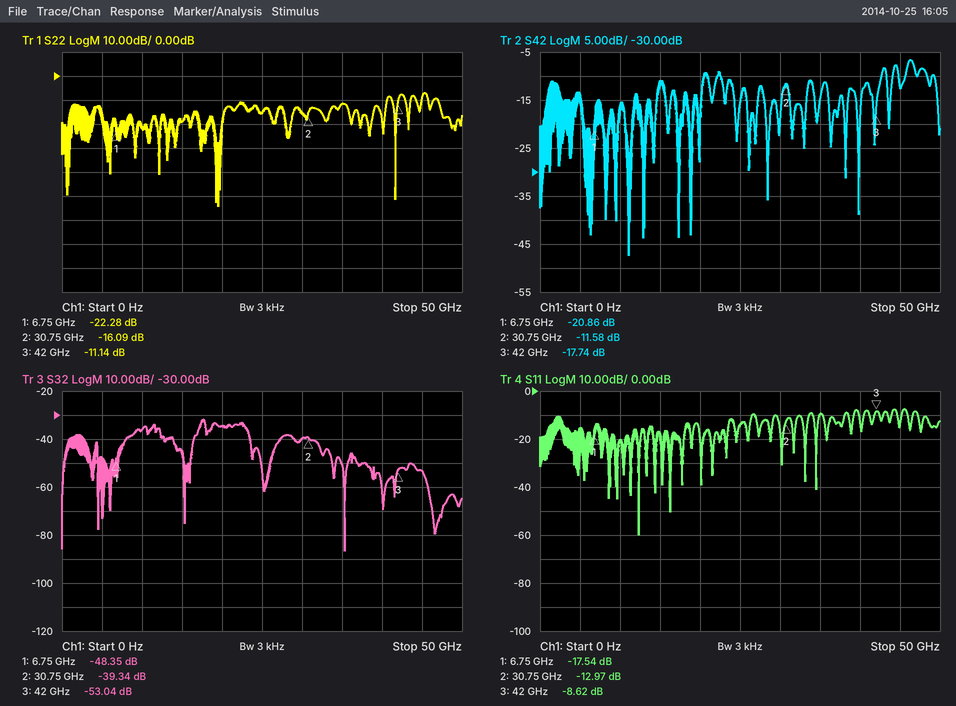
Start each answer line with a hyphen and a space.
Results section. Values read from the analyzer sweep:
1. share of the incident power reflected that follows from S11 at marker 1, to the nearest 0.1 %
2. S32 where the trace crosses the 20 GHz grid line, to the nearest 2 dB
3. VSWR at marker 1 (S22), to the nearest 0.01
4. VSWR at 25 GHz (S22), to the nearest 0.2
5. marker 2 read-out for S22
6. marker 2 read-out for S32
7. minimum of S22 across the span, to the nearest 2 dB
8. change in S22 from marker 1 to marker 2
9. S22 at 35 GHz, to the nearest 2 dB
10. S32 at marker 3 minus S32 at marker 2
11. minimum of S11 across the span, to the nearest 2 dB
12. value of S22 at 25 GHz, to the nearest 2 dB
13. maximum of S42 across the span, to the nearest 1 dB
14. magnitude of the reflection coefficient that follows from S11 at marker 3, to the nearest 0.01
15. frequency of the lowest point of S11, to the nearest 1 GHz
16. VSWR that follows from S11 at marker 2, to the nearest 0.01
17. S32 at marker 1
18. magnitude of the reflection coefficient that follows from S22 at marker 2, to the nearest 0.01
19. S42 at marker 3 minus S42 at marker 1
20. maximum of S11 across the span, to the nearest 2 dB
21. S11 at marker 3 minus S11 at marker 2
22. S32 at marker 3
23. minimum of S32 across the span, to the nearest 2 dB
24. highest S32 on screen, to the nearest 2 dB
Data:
- 1.8 %
- -34 dB
- 1.17
- 1.4
- -16.09 dB
- -39.34 dB
- -54 dB
- 6.19 dB
- -12 dB
- -13.70 dB
- -60 dB
- -16 dB
- -7 dB
- 0.37
- 12 GHz
- 1.58
- -48.35 dB
- 0.16
- 3.12 dB
- -8 dB
- 4.35 dB
- -53.04 dB
- -86 dB
- -32 dB
